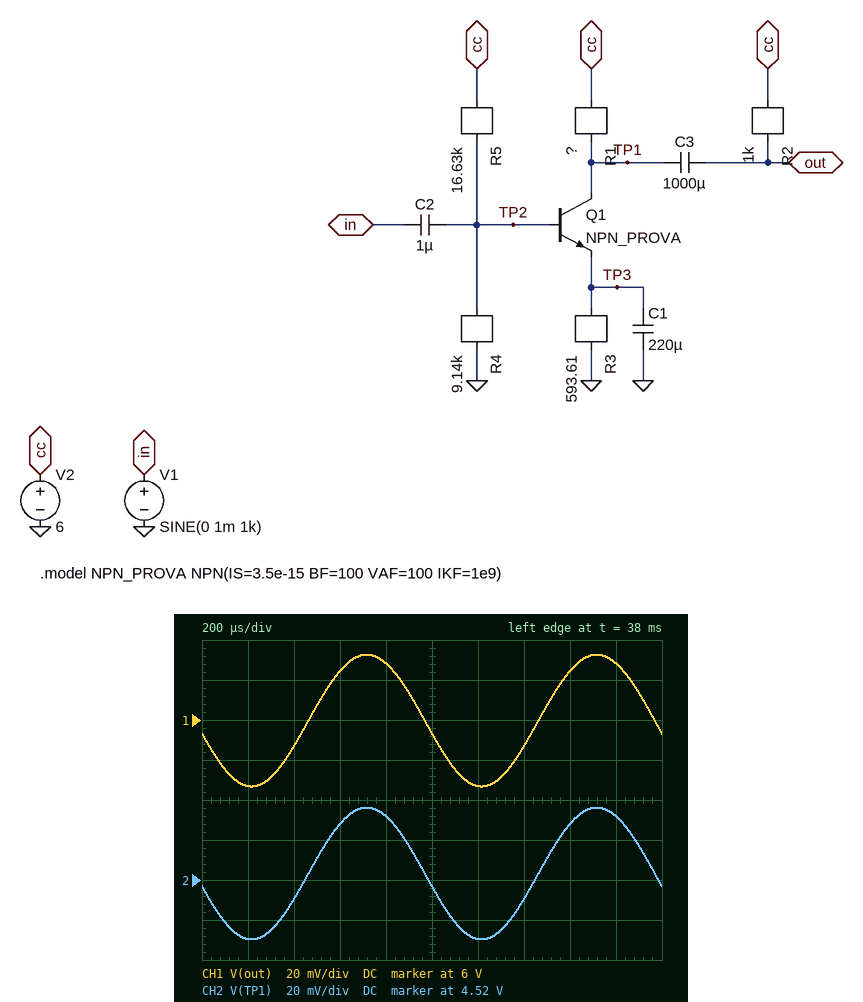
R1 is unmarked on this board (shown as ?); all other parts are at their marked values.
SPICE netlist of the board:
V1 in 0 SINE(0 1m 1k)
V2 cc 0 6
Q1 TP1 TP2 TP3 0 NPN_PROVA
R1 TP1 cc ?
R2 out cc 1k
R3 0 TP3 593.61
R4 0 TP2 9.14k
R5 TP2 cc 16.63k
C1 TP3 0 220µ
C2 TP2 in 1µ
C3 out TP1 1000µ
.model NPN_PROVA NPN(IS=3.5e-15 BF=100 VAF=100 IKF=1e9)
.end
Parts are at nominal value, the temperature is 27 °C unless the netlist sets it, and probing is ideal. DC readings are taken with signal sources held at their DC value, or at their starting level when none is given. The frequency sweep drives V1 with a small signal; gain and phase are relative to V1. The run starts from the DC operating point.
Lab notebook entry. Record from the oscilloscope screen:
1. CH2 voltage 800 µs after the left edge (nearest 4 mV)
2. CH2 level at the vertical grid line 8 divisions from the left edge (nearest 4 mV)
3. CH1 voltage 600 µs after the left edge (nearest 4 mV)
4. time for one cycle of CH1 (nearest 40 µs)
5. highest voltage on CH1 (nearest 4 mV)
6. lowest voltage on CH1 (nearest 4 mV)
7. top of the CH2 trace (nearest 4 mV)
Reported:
4.552 V
4.548 V
6.024 V
1.00 ms
6.032 V
5.968 V
4.556 V
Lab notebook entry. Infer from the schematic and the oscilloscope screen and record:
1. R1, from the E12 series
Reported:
680 Ω
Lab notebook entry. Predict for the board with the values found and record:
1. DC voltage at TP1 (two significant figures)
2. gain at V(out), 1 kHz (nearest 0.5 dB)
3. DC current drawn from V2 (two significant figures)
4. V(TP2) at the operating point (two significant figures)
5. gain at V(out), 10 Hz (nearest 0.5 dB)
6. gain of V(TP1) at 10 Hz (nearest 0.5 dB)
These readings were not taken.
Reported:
4.5 V
30.5 dB
2.4 mA
2.0 V
1.5 dB
1.5 dB
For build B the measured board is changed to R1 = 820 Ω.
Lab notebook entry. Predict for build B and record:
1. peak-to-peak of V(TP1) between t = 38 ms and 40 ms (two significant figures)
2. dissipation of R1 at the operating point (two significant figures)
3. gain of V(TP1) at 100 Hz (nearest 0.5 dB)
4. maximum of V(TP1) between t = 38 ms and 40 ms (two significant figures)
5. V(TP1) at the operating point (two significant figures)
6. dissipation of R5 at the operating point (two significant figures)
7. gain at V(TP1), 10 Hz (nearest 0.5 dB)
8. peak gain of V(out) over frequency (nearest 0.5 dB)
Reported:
73 mV
3.9 mW
24.0 dB
4.3 V
4.2 V
960 µW
2.5 dB
31.5 dB
